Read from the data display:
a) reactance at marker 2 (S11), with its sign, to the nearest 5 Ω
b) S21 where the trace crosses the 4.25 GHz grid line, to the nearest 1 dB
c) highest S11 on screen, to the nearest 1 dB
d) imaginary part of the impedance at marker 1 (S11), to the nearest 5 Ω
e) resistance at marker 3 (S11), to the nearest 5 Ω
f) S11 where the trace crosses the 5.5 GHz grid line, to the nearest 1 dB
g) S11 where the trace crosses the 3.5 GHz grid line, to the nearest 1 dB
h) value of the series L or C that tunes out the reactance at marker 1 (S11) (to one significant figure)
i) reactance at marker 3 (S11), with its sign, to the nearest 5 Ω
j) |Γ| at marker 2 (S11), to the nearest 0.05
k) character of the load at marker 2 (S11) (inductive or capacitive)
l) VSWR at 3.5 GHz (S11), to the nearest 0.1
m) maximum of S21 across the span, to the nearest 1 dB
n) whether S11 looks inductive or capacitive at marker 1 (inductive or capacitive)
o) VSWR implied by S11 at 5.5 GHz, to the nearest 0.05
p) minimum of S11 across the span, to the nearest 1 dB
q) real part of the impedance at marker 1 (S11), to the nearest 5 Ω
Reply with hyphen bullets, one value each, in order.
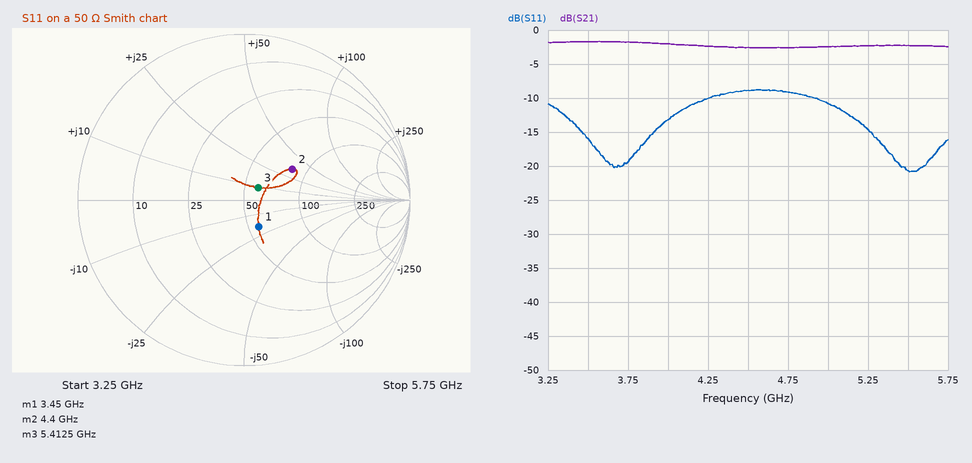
- +35 Ω
- -2 dB
- -9 dB
- -20 Ω
- 60 Ω
- -21 dB
- -16 dB
- 900 pH
- +10 Ω
- 0.35
- inductive
- 1.4
- -2 dB
- capacitive
- 1.20
- -21 dB
- 55 Ω
